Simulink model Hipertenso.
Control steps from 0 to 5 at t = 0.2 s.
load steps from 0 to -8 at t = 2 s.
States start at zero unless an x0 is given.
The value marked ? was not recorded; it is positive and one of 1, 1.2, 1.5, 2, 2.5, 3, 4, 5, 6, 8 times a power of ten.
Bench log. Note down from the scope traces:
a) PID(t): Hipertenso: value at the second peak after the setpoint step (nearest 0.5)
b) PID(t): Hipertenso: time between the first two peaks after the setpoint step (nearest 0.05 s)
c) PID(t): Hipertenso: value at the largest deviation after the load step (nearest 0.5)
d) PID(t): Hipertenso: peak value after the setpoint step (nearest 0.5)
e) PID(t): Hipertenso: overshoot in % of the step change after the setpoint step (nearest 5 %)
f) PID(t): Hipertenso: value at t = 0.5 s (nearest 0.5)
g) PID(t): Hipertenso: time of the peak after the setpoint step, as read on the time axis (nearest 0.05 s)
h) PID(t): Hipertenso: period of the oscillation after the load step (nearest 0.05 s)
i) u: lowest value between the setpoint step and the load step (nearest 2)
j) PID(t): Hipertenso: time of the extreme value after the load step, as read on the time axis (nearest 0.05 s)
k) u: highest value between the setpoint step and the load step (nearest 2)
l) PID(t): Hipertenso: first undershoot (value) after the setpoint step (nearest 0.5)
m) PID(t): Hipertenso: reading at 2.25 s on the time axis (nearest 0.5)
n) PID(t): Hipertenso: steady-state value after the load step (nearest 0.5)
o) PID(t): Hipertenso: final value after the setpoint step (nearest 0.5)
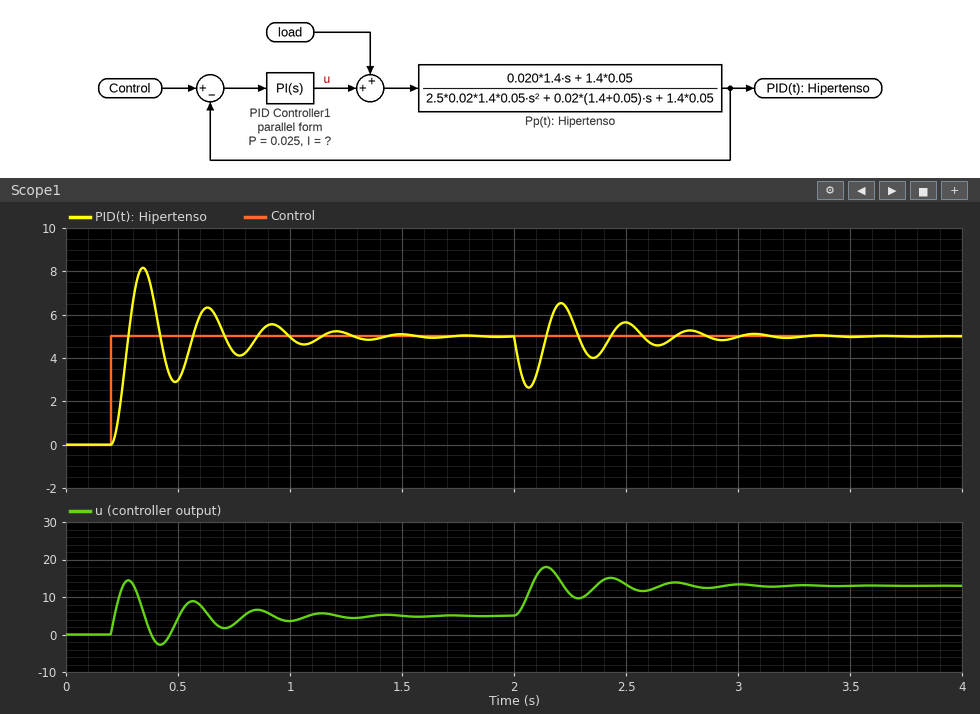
6.5
0.30 s
2.5
8.0
65 %
3.0
0.35 s
0.30 s
-2
2.05 s
14
3.0
6.0
5.0
5.0
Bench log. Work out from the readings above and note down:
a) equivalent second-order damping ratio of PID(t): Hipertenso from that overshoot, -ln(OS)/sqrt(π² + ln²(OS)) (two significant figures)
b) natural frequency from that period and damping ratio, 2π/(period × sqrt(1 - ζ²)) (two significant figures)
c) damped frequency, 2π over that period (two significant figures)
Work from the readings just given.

0.14
21 rad/s
21 rad/s
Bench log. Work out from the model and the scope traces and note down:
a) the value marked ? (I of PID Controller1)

60
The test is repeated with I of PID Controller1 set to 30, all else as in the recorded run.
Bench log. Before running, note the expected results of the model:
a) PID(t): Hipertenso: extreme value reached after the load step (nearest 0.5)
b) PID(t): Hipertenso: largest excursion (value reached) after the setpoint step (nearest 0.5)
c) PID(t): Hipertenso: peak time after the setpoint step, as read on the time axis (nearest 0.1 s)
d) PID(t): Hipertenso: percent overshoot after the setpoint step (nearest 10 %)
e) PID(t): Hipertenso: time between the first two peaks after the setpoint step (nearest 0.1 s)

2.0
7.5
0.4 s
50 %
0.4 s
